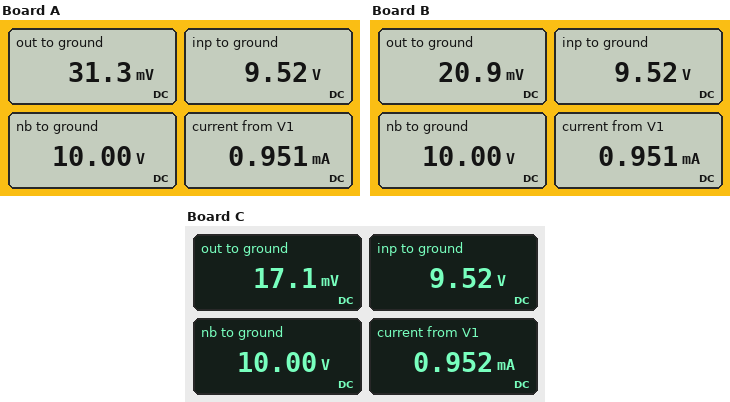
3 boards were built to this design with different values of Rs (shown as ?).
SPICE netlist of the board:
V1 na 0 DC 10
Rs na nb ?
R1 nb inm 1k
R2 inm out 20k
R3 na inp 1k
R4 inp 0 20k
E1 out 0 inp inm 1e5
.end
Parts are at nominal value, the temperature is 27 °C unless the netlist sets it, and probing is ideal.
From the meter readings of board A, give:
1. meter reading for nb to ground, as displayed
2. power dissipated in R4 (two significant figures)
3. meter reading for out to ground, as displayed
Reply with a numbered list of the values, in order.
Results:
1. 10.00 V
2. 4.5 mW
3. 31.3 mV
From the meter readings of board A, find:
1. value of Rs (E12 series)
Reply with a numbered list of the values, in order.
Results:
1. 3.3 Ω
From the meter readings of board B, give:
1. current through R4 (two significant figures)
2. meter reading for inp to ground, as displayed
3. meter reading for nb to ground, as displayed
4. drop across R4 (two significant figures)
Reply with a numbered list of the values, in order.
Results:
1. 480 µA
2. 9.52 V
3. 10.00 V
4. 9.5 V
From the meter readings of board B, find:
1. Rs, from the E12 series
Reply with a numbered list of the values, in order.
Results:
1. 2.2 Ω
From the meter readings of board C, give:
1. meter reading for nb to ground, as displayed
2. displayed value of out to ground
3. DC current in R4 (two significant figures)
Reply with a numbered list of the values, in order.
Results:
1. 10.00 V
2. 17.1 mV
3. 480 µA
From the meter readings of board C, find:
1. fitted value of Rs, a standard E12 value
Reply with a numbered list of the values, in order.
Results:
1. 1.8 Ω
